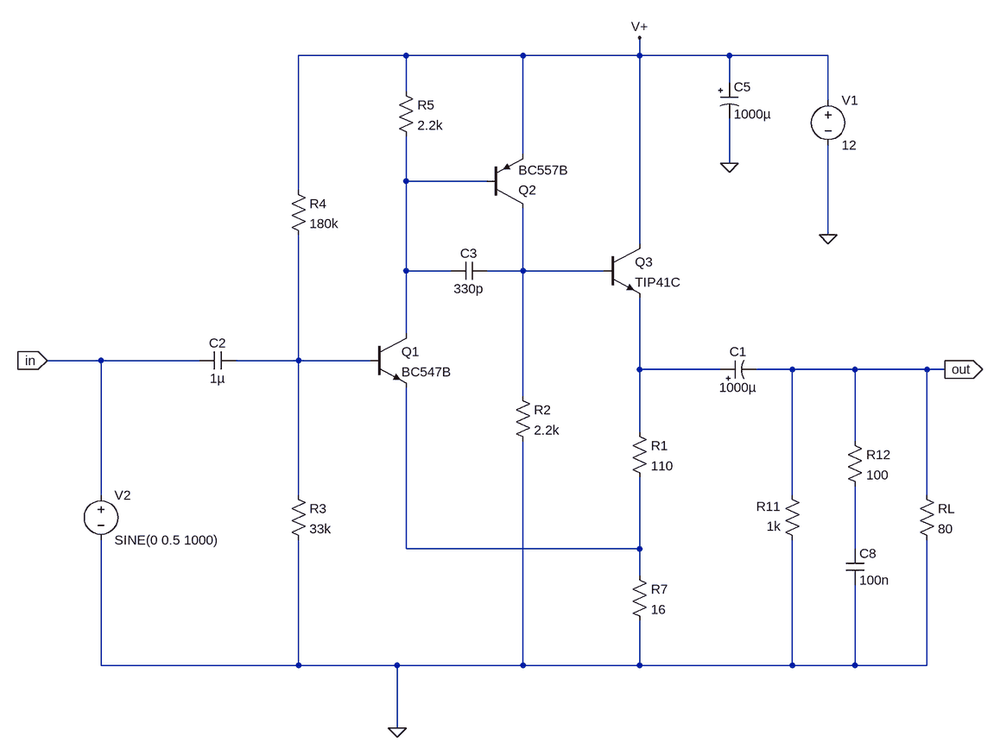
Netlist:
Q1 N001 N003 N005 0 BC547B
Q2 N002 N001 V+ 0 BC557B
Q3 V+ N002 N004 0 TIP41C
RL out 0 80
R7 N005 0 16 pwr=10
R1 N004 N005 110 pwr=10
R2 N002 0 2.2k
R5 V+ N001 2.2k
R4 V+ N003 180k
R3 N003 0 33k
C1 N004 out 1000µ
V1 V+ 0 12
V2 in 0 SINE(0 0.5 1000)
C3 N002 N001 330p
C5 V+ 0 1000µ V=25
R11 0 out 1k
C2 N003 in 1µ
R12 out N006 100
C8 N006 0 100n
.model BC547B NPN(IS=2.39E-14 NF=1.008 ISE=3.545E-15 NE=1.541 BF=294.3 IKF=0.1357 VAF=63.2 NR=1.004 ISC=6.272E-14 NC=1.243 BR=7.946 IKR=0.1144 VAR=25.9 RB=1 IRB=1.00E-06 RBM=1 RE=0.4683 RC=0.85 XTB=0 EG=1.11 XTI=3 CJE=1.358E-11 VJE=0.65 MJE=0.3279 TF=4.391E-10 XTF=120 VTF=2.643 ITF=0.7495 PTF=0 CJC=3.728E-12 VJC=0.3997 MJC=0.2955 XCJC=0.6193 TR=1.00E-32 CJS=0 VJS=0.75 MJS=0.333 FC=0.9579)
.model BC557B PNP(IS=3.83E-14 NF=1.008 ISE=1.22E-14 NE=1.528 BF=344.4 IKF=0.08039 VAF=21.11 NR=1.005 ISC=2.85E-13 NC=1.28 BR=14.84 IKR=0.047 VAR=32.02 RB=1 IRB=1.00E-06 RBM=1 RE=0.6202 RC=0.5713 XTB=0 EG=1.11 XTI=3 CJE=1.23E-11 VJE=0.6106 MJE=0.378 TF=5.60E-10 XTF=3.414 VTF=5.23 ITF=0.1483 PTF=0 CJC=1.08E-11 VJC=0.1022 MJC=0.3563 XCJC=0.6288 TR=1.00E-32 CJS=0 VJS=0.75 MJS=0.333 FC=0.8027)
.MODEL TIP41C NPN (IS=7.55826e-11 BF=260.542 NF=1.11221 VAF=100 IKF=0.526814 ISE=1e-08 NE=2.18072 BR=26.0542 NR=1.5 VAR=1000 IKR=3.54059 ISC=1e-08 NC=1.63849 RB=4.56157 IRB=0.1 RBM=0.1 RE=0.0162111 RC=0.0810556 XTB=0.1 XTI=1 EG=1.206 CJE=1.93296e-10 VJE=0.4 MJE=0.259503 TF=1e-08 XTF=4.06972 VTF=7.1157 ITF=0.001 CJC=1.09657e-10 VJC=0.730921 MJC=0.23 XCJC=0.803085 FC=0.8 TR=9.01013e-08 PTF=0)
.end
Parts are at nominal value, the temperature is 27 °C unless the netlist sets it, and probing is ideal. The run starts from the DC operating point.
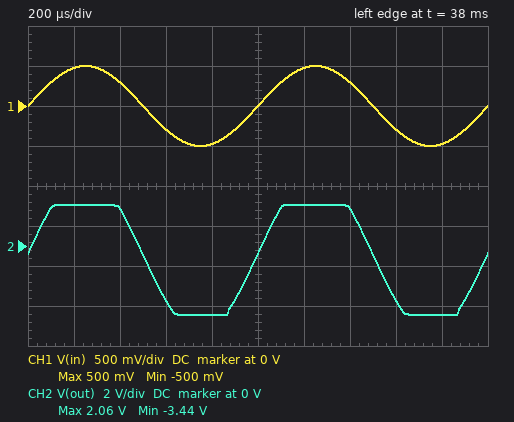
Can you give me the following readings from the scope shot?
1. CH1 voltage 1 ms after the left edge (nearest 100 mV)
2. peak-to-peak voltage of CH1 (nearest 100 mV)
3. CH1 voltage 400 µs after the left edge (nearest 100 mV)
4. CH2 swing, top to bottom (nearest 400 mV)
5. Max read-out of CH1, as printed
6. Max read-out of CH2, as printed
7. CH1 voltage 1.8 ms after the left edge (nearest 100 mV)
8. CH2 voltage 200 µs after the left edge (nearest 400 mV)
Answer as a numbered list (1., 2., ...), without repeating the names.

1. 0 V
2. 1.0 V
3. 300 mV
4. 5.6 V
5. 500 mV
6. 2.06 V
7. -500 mV
8. 2.0 V
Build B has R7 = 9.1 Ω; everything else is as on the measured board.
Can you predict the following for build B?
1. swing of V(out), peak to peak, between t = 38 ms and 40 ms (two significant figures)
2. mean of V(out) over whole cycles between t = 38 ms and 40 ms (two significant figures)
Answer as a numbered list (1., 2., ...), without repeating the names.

1. 4.9 V
2. -1.5 V
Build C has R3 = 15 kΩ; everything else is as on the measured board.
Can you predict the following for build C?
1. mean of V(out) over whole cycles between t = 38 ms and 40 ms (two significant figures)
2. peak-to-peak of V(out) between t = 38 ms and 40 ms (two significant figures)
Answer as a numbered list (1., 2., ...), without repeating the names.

1. 590 mV
2. 4.6 V
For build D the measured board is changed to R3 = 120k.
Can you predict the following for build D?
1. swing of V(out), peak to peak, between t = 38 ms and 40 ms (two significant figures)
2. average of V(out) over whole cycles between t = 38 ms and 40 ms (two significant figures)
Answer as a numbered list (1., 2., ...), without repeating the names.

1. 3.3 V
2. -600 mV
